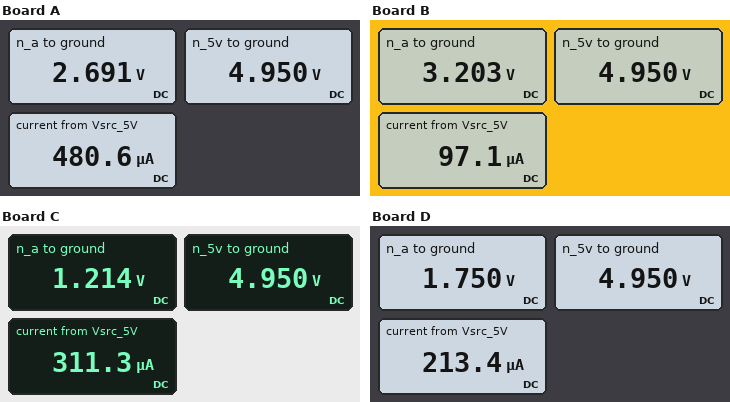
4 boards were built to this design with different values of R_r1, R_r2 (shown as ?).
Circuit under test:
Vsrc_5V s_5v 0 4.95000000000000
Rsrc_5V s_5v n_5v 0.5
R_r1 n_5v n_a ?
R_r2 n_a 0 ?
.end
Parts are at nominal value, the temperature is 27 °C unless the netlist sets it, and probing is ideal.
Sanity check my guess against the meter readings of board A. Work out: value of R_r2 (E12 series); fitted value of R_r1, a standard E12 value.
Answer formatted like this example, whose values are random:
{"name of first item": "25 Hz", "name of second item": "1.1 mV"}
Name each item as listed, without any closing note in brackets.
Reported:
{"value of R_r2": "5.6 kΩ", "fitted value of R_r1, a standard E12 value": "4.7 kΩ"}
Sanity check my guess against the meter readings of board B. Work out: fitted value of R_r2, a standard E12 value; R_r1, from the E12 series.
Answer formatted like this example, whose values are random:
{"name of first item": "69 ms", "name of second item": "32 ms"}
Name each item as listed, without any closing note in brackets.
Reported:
{"fitted value of R_r2, a standard E12 value": "33 kΩ", "R_r1, from the E12 series": "18 kΩ"}
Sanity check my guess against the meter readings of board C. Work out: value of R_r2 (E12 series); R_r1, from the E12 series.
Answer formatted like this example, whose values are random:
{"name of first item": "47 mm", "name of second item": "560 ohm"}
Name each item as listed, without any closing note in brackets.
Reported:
{"value of R_r2": "3.9 kΩ", "R_r1, from the E12 series": "12 kΩ"}
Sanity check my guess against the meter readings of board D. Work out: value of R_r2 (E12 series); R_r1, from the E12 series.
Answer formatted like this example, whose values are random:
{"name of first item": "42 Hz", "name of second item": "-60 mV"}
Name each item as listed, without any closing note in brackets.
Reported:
{"value of R_r2": "8.2 kΩ", "R_r1, from the E12 series": "15 kΩ"}
